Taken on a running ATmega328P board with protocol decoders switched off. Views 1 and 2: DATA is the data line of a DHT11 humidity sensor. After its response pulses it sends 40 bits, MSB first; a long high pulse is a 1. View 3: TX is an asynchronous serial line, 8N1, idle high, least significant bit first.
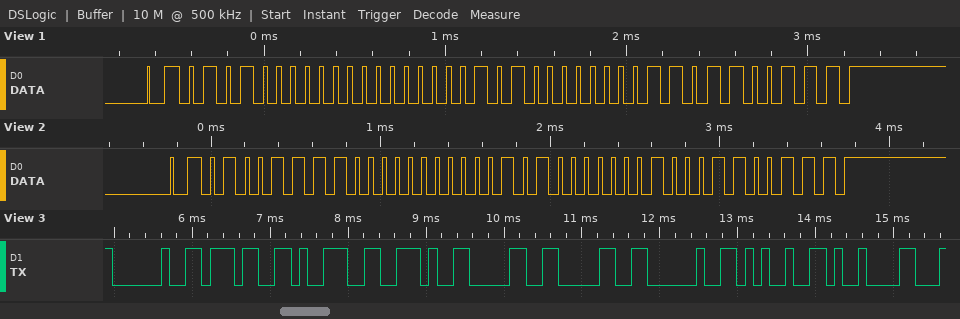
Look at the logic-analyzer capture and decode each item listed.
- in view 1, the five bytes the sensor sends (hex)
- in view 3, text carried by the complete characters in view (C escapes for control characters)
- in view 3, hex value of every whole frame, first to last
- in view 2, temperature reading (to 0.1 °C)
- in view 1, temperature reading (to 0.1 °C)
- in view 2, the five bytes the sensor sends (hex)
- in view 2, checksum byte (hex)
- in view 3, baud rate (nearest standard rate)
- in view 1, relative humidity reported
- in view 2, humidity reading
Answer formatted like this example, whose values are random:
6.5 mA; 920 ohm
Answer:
50 00 14 03 67; " 79.00 %\t"; 20 37 39 2E 30 30 20 25 09; 20.4 °C; 20.3 °C; 4F 00 14 04 67; 0x67; 9600 baud; 80 %; 79 %
